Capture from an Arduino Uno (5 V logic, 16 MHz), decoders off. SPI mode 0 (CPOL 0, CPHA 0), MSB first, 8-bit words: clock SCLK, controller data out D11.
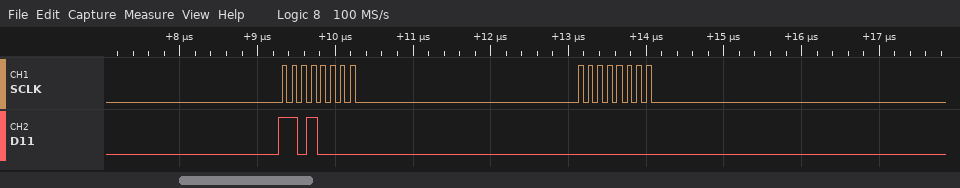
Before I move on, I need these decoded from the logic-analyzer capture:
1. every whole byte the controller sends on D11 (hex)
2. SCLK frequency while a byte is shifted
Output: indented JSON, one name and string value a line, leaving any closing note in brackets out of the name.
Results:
{
  "every whole byte the controller sends on D11": "0xD0 0x00",
  "SCLK frequency while a byte is shifted": "8 MHz"
}
